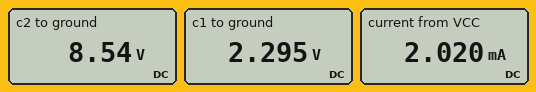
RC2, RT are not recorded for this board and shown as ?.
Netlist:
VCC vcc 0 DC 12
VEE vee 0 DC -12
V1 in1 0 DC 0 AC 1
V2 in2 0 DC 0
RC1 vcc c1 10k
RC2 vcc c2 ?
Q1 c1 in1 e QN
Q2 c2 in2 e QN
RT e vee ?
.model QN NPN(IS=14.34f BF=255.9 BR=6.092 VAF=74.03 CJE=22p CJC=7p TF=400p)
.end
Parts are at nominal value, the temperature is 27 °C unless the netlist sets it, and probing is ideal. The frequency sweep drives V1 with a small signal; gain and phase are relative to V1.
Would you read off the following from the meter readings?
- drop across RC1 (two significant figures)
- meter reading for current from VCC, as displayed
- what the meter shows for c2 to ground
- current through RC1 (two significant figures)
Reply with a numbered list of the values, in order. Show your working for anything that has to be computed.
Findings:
1. 12 V - 2.295 V = 9.7 V
2. 2.020 mA
3. 8.54 V
4. (12 V - 2.295 V) / 10 kΩ = 970 µA
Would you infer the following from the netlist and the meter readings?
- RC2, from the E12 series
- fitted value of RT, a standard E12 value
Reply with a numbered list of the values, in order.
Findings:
1. 3.3 kΩ
2. 5.6 kΩ
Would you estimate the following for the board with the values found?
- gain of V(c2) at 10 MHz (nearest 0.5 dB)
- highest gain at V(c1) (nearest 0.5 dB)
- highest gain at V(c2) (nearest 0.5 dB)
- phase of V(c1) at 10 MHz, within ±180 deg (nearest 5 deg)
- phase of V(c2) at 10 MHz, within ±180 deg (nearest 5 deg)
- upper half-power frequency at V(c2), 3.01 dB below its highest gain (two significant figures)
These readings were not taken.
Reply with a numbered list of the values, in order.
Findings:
1. 34.5 dB
2. 45.0 dB
3. 35.5 dB
4. 110 deg
5. -30 deg
6. 18 MHz
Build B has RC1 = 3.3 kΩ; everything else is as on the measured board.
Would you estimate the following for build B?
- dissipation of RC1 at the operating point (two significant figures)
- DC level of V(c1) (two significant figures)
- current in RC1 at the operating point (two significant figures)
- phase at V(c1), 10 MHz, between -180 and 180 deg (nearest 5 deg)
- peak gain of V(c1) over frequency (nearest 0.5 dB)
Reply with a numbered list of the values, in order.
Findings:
1. 3.4 mW
2. 8.7 V
3. 1.0 mA
4. 150 deg
5. 36.0 dB
